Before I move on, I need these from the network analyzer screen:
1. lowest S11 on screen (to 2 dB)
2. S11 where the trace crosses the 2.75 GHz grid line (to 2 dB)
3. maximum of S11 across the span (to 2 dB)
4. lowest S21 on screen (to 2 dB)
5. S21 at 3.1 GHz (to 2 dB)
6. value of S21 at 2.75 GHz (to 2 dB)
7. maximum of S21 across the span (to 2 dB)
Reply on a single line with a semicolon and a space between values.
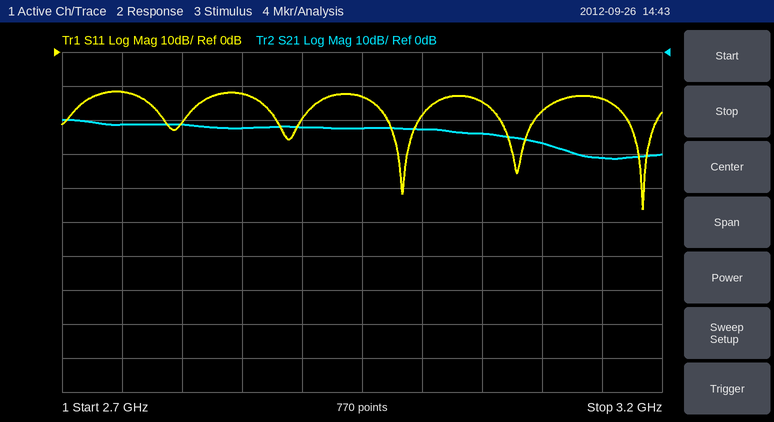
-46 dB; -12 dB; -12 dB; -32 dB; -26 dB; -22 dB; -20 dB
